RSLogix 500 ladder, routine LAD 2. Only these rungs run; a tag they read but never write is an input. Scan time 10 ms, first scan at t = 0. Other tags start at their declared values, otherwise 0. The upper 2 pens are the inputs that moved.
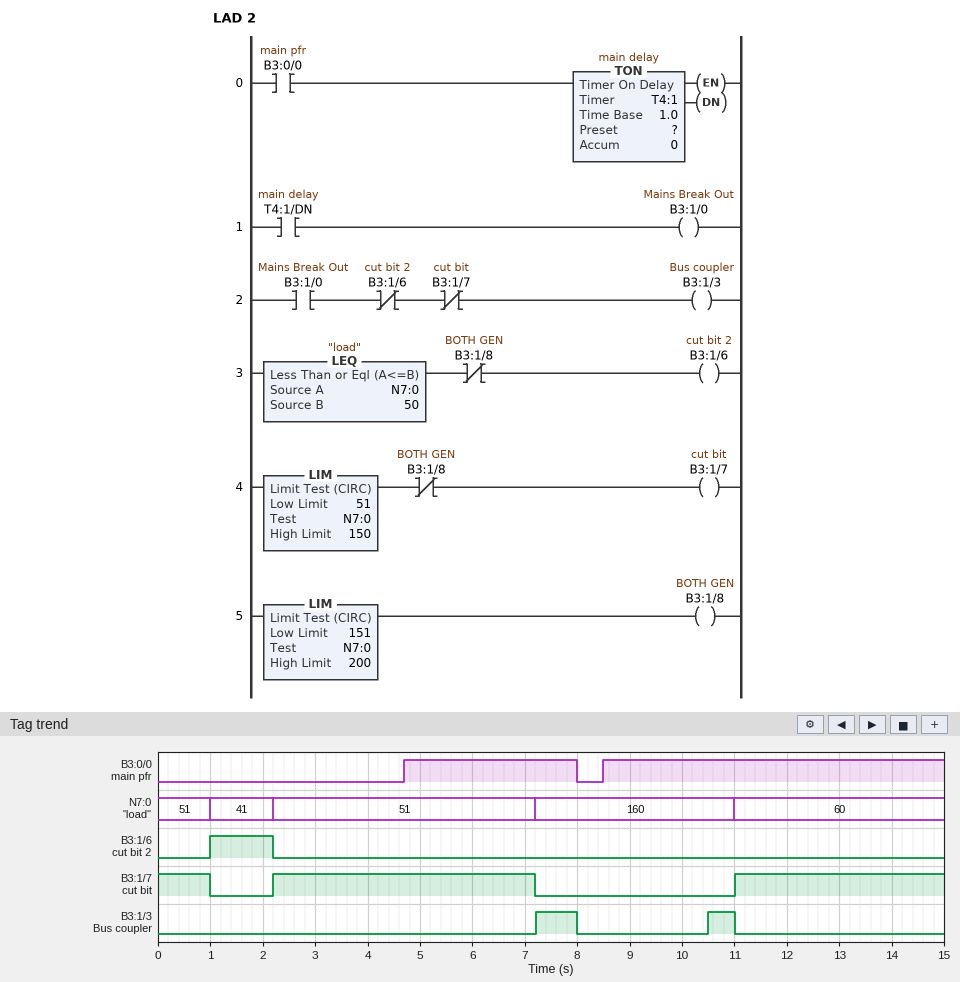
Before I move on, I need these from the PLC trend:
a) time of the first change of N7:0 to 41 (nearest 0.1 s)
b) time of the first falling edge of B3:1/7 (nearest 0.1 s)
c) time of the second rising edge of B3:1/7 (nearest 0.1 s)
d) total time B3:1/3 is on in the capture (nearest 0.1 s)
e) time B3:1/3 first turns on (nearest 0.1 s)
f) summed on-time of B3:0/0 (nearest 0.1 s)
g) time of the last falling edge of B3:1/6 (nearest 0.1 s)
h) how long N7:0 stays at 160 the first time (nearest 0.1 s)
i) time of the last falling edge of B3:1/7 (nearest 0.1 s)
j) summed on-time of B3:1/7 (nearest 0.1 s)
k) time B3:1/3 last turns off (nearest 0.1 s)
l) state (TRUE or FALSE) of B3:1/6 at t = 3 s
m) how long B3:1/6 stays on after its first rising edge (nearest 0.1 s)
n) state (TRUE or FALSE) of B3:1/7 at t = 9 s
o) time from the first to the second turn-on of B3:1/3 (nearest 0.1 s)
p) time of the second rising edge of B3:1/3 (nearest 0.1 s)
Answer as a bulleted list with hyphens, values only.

- 1.0 s
- 1.0 s
- 11.0 s
- 1.3 s
- 7.2 s
- 9.8 s
- 2.2 s
- 3.8 s
- 7.2 s
- 10.0 s
- 11.0 s
- FALSE
- 1.2 s
- FALSE
- 3.3 s
- 10.5 s
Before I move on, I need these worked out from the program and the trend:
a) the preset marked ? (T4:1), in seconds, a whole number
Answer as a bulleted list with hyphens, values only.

- 2 s
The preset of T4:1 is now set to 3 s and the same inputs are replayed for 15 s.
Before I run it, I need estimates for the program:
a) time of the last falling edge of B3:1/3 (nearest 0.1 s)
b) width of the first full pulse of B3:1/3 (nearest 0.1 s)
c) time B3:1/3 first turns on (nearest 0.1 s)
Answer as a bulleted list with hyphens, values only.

- 8.0 s
- 0.3 s
- 7.7 s
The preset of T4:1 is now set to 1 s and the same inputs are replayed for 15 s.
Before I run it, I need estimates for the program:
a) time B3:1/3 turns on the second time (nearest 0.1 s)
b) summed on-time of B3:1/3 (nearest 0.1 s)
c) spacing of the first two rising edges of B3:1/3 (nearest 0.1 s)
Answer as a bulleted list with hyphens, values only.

- 9.5 s
- 2.3 s
- 2.3 s
